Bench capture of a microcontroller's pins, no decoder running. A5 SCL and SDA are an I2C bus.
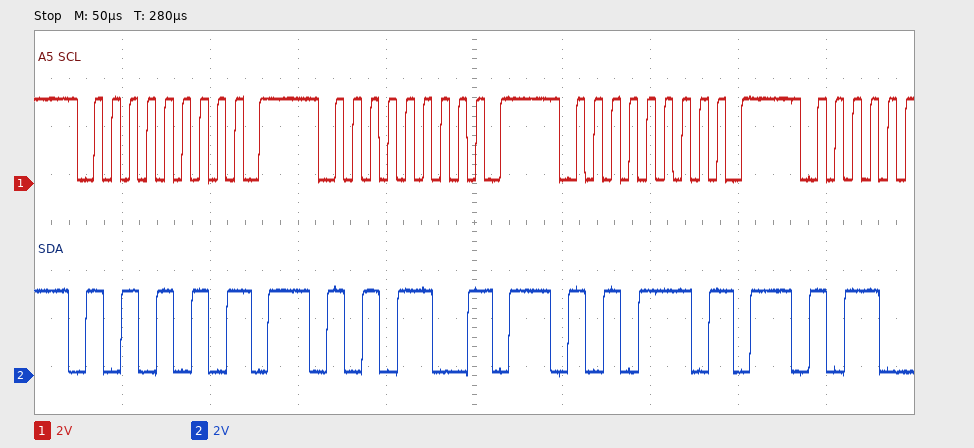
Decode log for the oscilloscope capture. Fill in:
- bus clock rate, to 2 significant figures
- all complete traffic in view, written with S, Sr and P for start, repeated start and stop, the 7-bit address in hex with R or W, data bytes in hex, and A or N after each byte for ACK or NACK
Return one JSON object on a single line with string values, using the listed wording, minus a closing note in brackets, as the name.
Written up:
{"bus clock rate, to 2 significant figures": "100 kHz", "all complete traffic in view, written with S, Sr and P for start, repeated start and stop, the 7-bit address in hex with R or W, data bytes in hex, and A or N after each byte for ACK or NACK": "S 55W N P S 56W N P S 57W N P"}
